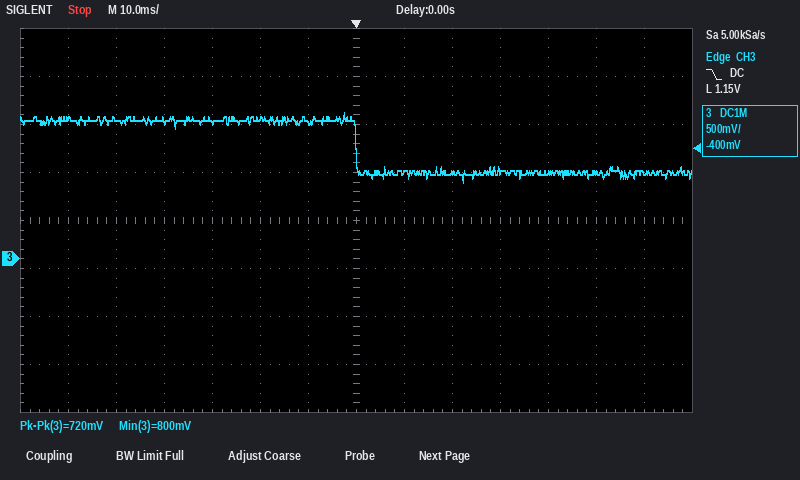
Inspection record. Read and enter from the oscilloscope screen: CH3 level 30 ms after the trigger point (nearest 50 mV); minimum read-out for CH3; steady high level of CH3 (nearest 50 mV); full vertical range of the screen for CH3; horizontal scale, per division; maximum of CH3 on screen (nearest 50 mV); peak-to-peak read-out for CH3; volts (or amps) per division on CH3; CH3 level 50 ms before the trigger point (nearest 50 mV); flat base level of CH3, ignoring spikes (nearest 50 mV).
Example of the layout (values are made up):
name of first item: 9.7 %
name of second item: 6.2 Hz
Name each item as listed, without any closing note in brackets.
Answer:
CH3 level 30 ms after the trigger point: 900 mV
minimum read-out for CH3: 800 mV
steady high level of CH3: 1.45 V
full vertical range of the screen for CH3: 4 V
horizontal scale, per division: 10 ms
maximum of CH3 on screen: 1.50 V
peak-to-peak read-out for CH3: 720 mV
volts (or amps) per division on CH3: 500 mV
CH3 level 50 ms before the trigger point: 1.45 V
flat base level of CH3, ignoring spikes: 900 mV
